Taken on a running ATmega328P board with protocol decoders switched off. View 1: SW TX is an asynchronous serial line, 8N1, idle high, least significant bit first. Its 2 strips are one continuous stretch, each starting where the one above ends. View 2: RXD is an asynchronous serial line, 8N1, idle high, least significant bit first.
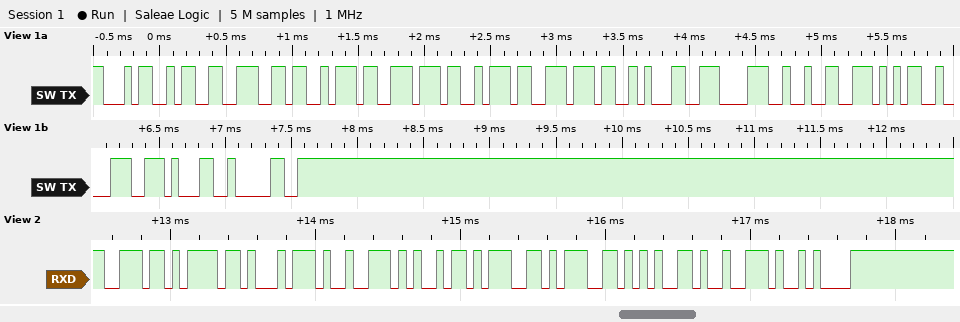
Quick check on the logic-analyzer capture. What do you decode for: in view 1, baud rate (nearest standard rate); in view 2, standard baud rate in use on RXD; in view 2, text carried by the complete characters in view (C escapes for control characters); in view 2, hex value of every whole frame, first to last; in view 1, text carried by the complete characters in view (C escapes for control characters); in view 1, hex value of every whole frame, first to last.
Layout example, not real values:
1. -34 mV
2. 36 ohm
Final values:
1. 19200 baud
2. 19200 baud
3. "notrigger\n"
4. 6E 6F 74 72 69 67 67 65 72 0A
5. "43677771825810"
6. 34 33 36 37 37 37 37 31 38 32 35 38 31 30
